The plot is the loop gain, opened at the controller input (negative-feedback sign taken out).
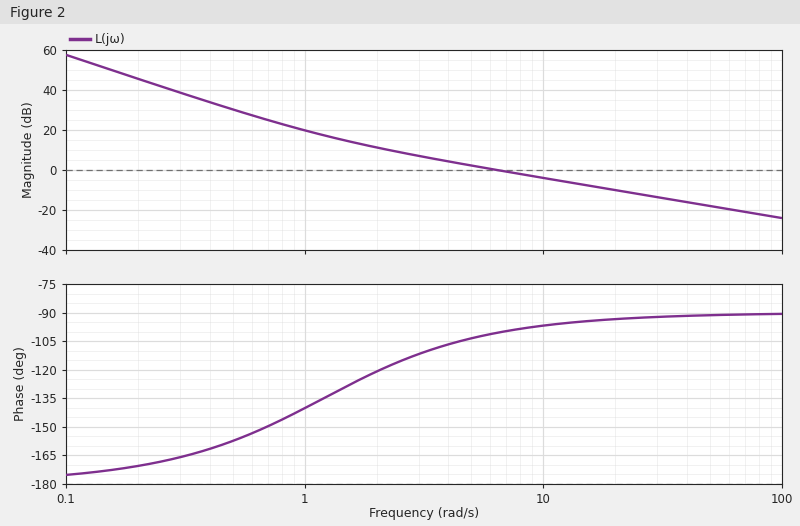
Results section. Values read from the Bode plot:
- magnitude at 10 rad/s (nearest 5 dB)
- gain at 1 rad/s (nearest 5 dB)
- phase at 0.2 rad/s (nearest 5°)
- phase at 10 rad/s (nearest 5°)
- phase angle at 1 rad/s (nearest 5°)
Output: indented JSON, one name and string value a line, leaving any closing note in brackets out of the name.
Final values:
{
  "magnitude at 10 rad/s": "-5 dB",
  "gain at 1 rad/s": "20 dB",
  "phase at 0.2 rad/s": "-170°",
  "phase at 10 rad/s": "-95°",
  "phase angle at 1 rad/s": "-140°"
}
